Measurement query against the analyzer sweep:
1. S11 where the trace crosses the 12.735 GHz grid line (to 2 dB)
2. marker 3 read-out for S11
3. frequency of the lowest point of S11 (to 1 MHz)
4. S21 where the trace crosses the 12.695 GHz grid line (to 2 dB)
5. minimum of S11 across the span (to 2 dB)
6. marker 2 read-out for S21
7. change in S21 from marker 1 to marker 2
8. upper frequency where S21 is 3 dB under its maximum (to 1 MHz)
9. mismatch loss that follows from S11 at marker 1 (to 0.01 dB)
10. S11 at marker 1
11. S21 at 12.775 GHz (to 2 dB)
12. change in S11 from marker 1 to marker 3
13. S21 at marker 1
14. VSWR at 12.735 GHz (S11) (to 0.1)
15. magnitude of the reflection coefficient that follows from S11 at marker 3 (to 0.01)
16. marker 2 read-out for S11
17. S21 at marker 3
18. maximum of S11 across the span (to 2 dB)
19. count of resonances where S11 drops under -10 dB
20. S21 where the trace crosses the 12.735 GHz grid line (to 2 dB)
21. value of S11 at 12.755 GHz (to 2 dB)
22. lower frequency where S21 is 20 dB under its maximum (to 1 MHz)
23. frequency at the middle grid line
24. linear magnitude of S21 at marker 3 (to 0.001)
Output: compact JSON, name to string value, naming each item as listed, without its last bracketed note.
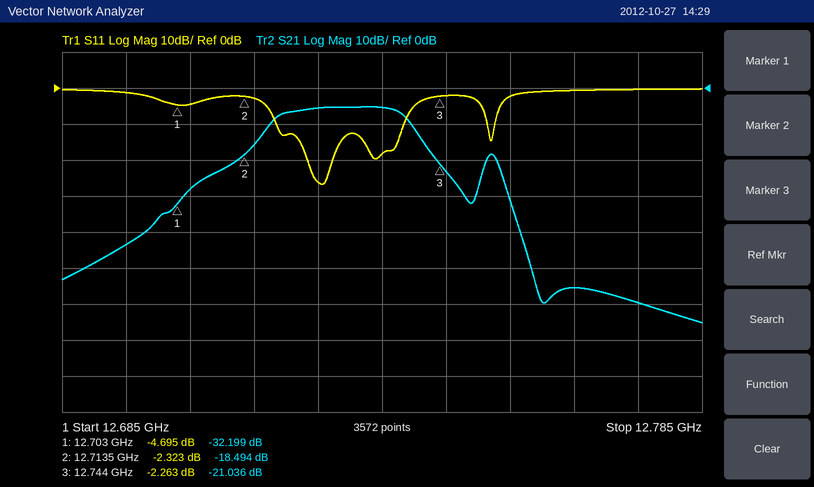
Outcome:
{"S11 where the trace crosses the 12.735 GHz grid line": "-18 dB", "marker 3 read-out for S11": "-2.263 dB", "frequency of the lowest point of S11": "12.726 GHz", "S21 where the trace crosses the 12.695 GHz grid line": "-44 dB", "minimum of S11 across the span": "-26 dB", "marker 2 read-out for S21": "-18.494 dB", "change in S21 from marker 1 to marker 2": "13.705 dB", "upper frequency where S21 is 3 dB under its maximum": "12.739 GHz", "mismatch loss that follows from S11 at marker 1": "1.80 dB", "S11 at marker 1": "-4.695 dB", "S21 at 12.775 GHz": "-60 dB", "change in S11 from marker 1 to marker 3": "2.432 dB", "S21 at marker 1": "-32.199 dB", "VSWR at 12.735 GHz (S11)": "1.3", "magnitude of the reflection coefficient that follows from S11 at marker 3": "0.77", "marker 2 read-out for S11": "-2.323 dB", "S21 at marker 3": "-21.036 dB", "maximum of S11 across the span": "0 dB", "count of resonances where S11 drops under -10 dB": "3", "S21 where the trace crosses the 12.735 GHz grid line": "-6 dB", "value of S11 at 12.755 GHz": "-2 dB", "lower frequency where S21 is 20 dB under its maximum": "12.707 GHz", "frequency at the middle grid line": "12.735 GHz", "linear magnitude of S21 at marker 3": "0.089"}
